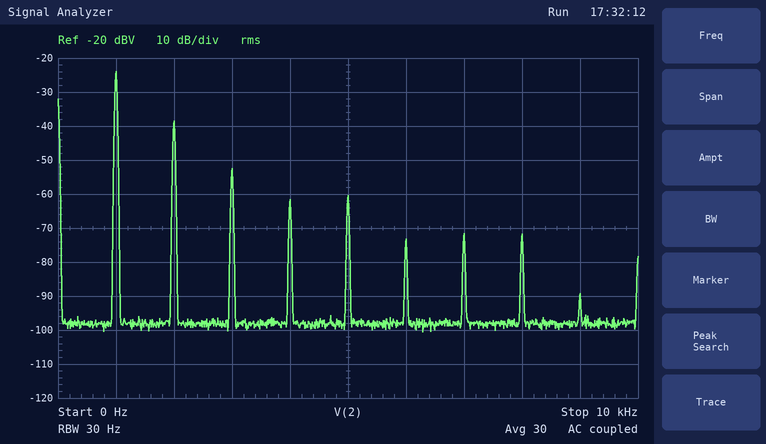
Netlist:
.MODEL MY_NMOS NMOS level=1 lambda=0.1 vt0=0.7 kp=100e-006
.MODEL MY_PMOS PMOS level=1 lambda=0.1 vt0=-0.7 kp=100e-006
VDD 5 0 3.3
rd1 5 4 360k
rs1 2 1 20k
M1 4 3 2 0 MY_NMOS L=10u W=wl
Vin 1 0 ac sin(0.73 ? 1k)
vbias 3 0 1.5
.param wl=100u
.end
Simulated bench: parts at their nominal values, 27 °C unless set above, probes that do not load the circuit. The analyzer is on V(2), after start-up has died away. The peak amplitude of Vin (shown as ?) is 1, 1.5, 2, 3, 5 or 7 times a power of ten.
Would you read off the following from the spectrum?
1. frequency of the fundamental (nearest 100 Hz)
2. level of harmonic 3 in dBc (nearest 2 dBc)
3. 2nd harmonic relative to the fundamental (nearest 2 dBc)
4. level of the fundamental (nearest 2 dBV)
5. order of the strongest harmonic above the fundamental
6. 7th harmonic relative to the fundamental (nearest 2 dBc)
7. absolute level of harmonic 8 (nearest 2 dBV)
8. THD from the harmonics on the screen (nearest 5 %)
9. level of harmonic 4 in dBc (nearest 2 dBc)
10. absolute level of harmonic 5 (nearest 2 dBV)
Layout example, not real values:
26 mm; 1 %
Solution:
1.0 kHz; -28 dBc; -14 dBc; -24 dBV; 2; -48 dBc; -72 dBV; 20 %; -38 dBc; -60 dBV
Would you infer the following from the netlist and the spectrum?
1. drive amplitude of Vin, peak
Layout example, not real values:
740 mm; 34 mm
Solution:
150 mV
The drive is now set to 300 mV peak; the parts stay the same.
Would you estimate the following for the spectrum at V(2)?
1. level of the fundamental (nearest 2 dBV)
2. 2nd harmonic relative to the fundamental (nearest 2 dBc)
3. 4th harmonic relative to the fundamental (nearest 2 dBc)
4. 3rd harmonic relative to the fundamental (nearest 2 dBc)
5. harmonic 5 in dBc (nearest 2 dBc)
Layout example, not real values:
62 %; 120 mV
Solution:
-16 dBV; -20 dBc; -26 dBc; -24 dBc; -42 dBc
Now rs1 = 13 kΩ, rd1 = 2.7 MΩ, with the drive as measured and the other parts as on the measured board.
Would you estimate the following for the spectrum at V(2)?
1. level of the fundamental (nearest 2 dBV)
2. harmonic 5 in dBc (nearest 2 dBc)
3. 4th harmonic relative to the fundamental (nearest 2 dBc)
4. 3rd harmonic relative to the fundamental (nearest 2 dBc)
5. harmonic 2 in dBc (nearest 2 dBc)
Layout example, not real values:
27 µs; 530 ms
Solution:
-20 dBV; -50 dBc; -40 dBc; -38 dBc; -38 dBc
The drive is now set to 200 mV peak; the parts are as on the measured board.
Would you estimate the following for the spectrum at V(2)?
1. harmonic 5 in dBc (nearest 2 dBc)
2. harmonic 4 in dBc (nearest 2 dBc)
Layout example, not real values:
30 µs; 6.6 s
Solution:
-40 dBc; -30 dBc
